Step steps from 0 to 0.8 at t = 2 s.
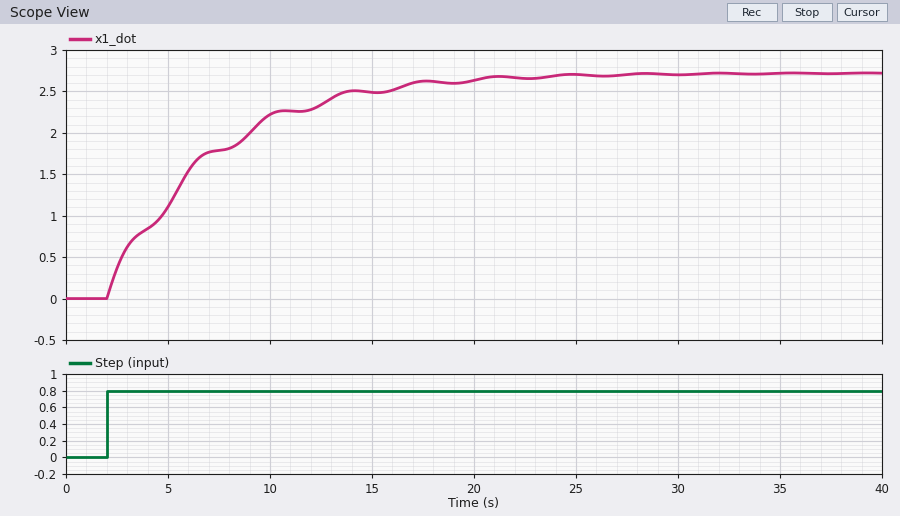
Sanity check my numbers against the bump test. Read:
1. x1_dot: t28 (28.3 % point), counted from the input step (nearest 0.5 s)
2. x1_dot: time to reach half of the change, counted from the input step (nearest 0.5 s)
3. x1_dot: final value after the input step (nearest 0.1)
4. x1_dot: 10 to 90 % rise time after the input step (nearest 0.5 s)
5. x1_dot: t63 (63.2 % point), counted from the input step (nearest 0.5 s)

1.5 s
3.5 s
2.7
11.0 s
4.5 s
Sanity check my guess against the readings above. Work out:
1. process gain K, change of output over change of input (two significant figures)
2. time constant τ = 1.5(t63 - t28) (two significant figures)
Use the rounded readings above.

3.4
4.5 s
